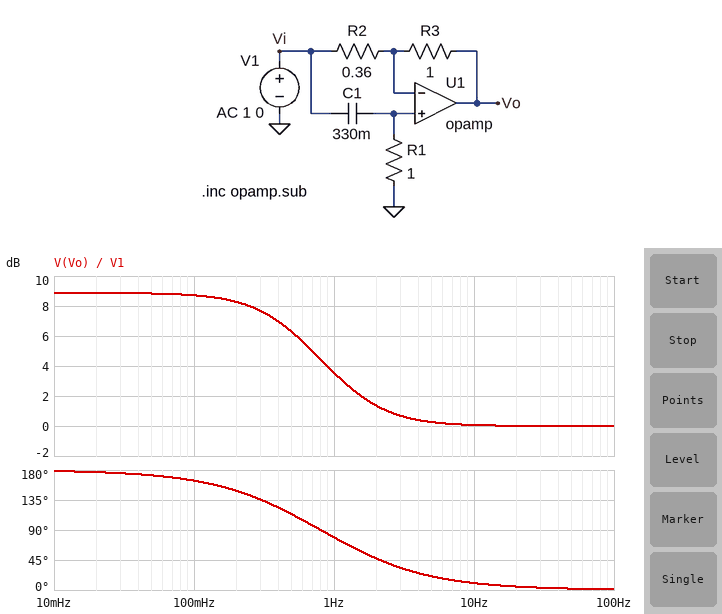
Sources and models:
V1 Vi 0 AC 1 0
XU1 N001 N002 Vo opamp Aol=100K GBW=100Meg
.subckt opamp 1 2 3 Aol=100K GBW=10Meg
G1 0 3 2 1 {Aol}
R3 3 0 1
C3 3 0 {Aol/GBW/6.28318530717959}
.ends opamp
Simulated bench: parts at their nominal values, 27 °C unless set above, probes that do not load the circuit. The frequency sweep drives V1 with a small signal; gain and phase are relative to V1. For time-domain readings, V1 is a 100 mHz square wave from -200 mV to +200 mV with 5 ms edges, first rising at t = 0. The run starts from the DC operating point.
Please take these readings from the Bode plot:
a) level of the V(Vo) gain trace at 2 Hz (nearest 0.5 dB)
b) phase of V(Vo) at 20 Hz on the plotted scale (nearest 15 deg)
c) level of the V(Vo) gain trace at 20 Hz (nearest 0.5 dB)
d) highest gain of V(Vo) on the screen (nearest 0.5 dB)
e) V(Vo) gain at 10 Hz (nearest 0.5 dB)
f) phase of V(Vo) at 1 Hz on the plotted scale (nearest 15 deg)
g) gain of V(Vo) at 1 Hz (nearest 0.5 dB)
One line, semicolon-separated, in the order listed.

1.5 dB; 0 deg; 0 dB; 9.0 dB; 0 dB; 75 deg; 3.5 dB
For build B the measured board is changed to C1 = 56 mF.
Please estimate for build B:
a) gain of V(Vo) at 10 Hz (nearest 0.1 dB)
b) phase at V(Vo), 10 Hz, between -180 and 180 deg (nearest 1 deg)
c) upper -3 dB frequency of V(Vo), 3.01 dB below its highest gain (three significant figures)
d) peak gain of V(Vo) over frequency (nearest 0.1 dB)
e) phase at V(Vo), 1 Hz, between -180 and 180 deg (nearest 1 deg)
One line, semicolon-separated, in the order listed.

1.8 dB; 54 deg; 3.30 Hz; 8.9 dB; 153 deg
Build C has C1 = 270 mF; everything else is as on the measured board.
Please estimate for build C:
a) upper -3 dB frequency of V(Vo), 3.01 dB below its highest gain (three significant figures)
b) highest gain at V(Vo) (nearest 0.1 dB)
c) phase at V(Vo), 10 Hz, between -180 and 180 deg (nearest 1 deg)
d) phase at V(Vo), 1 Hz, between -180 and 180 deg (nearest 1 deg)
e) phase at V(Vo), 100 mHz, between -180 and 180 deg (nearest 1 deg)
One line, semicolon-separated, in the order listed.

685 mHz; 8.9 dB; 13 deg; 89 deg; 167 deg
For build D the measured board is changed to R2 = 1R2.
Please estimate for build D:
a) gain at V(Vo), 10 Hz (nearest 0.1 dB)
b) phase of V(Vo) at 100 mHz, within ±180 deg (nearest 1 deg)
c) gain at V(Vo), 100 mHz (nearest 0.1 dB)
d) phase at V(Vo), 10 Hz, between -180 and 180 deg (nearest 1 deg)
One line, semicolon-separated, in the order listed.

0 dB; 154 deg; -1.5 dB; 5 deg
